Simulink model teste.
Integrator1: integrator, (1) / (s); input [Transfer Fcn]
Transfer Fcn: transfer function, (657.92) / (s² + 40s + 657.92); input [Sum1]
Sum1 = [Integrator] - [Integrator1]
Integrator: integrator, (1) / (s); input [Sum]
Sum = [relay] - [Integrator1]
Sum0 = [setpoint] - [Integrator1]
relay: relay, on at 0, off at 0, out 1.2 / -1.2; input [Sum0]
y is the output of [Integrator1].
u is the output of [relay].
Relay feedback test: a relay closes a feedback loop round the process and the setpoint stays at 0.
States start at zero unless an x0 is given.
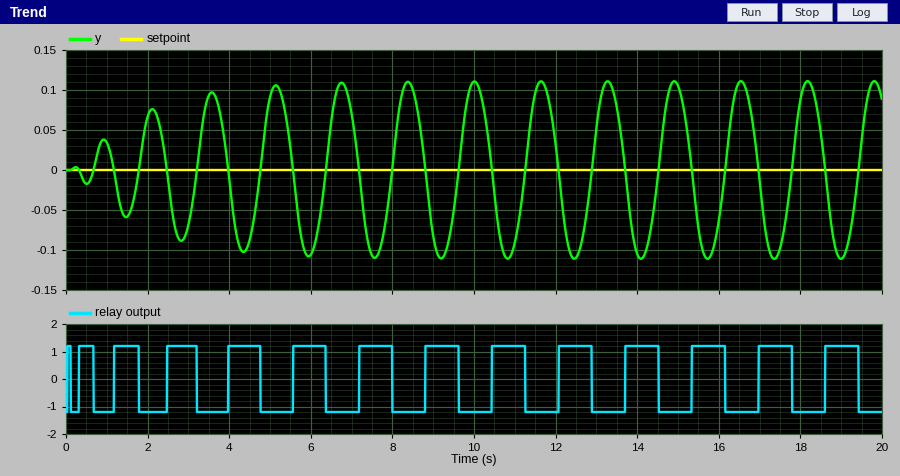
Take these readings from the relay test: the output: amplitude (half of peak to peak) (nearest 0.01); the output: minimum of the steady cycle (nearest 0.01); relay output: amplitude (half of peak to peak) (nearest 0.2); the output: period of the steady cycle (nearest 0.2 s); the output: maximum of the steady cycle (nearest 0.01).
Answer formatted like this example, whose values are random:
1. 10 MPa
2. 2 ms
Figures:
1. 0.11
2. -0.11
3. 1.2
4. 1.6 s
5. 0.11
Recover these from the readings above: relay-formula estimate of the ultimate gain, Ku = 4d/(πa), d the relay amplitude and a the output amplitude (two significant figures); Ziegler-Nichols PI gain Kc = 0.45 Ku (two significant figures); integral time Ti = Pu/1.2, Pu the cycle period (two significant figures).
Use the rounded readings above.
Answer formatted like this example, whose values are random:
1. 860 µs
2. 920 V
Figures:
1. 14
2. 6.3
3. 1.3 s
